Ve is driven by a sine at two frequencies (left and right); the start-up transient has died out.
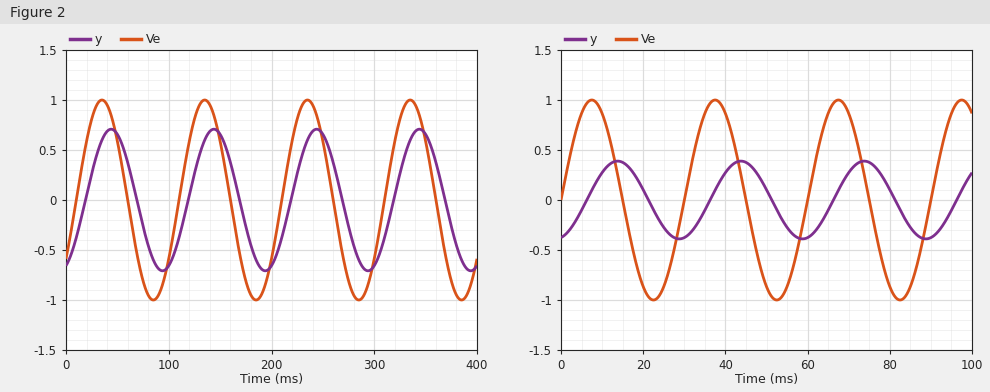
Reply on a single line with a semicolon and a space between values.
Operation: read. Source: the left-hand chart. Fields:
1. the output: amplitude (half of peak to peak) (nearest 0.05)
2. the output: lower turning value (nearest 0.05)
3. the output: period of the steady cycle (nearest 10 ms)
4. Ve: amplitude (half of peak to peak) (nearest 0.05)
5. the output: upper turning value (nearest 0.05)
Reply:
0.70; -0.70; 100 ms; 1.00; 0.70
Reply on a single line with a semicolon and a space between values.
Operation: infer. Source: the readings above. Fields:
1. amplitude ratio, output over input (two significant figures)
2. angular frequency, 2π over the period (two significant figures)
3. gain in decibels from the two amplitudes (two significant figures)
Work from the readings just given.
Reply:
0.70; 0.063 rad/ms; -3.1 dB
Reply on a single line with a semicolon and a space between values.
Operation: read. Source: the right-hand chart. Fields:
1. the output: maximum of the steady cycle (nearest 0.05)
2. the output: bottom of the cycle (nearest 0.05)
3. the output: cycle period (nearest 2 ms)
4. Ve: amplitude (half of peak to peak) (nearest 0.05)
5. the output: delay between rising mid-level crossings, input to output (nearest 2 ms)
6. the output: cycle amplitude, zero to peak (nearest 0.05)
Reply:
0.40; -0.40; 30 ms; 1.00; 6 ms; 0.40
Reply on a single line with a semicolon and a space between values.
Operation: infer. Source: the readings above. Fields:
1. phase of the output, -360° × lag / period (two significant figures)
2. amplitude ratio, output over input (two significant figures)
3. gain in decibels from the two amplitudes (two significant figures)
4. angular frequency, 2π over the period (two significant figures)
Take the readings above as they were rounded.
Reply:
-72°; 0.40; -8.0 dB; 0.21 rad/ms
